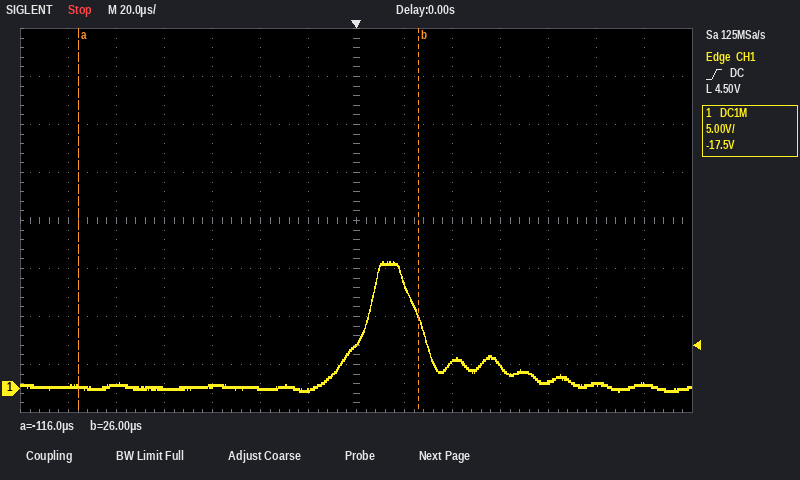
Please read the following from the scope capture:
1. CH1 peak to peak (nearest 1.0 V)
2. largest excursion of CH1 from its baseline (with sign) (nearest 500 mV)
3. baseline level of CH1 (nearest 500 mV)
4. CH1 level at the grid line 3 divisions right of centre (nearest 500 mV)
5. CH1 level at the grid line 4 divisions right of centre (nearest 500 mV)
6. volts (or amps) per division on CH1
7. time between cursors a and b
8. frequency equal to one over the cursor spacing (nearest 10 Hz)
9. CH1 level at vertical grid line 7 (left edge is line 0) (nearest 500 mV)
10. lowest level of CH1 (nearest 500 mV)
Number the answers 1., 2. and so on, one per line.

1. 14.0 V
2. +13.0 V
3. 0.0 V
4. 2.5 V
5. 500 mV
6. 5 V
7. 142 µs
8. 7.04 kHz
9. 4.5 V
10. -500 mV
